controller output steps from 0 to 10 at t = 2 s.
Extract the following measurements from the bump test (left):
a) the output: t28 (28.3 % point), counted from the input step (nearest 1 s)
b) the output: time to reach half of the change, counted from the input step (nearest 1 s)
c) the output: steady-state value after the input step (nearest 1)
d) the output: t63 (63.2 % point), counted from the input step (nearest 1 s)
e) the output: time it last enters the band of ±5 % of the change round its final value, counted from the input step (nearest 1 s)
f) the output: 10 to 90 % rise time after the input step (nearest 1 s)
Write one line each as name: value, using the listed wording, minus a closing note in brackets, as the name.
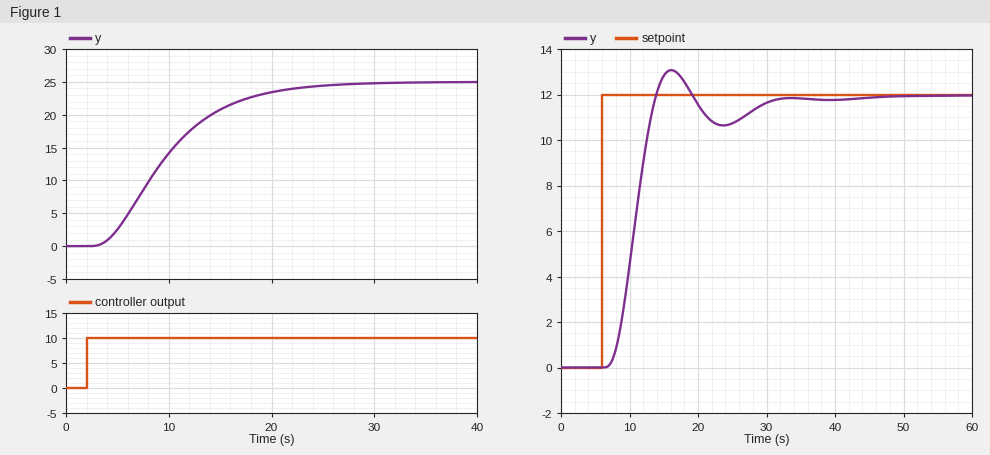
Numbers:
the output: t28 (28.3 % point), counted from the input step: 5 s
the output: time to reach half of the change, counted from the input step: 7 s
the output: steady-state value after the input step: 25
the output: t63 (63.2 % point), counted from the input step: 9 s
the output: time it last enters the band of ±5 % of the change round its final value, counted from the input step: 19 s
the output: 10 to 90 % rise time after the input step: 13 s
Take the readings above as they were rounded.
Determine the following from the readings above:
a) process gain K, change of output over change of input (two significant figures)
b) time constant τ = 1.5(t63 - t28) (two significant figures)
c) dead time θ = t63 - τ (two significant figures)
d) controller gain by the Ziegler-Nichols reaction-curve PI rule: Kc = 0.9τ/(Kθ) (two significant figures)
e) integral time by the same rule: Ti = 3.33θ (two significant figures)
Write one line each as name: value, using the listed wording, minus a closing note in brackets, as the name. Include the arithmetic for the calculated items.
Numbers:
process gain K, change of output over change of input: (25 - 0) / 10 = 2.5
time constant τ = 1.5(t63 - t28): 1.5 × (9 - 5) = 6.0 s
dead time θ = t63 - τ: 9 - 6 = 3.0 s
controller gain by the Ziegler-Nichols reaction-curve PI rule: Kc = 0.9τ/(Kθ): 0.9 × 6 / (2.5 × 3) = 0.72
integral time by the same rule: Ti = 3.33θ: 3.33 × 3 = 10.0 s
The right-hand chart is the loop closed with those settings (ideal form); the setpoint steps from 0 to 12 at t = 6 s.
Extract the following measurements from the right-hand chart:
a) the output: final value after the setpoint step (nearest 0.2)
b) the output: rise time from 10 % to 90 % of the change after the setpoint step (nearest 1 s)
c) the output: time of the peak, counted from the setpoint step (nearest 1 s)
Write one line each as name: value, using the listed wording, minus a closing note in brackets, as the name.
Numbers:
the output: final value after the setpoint step: 12.0
the output: rise time from 10 % to 90 % of the change after the setpoint step: 5 s
the output: time of the peak, counted from the setpoint step: 10 s
